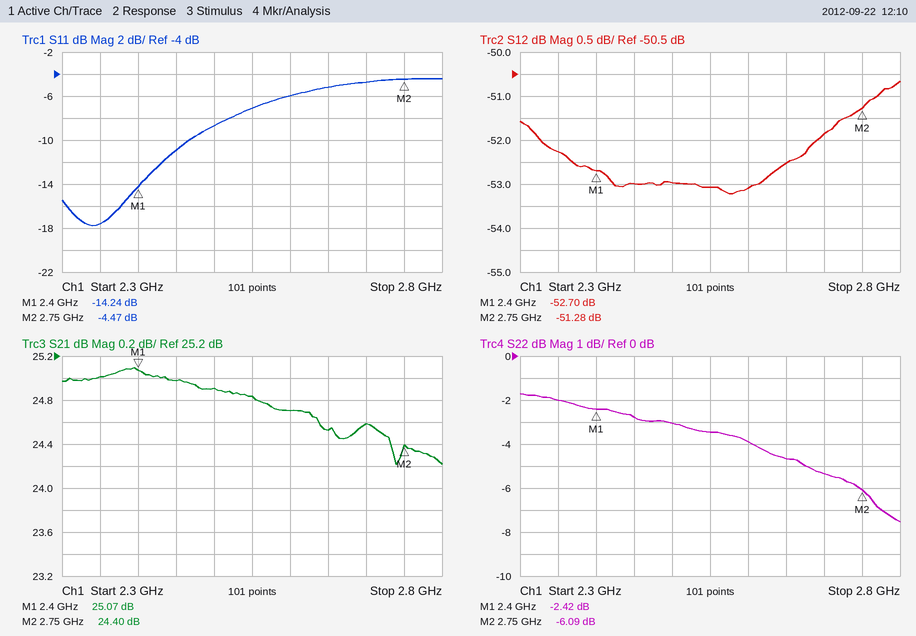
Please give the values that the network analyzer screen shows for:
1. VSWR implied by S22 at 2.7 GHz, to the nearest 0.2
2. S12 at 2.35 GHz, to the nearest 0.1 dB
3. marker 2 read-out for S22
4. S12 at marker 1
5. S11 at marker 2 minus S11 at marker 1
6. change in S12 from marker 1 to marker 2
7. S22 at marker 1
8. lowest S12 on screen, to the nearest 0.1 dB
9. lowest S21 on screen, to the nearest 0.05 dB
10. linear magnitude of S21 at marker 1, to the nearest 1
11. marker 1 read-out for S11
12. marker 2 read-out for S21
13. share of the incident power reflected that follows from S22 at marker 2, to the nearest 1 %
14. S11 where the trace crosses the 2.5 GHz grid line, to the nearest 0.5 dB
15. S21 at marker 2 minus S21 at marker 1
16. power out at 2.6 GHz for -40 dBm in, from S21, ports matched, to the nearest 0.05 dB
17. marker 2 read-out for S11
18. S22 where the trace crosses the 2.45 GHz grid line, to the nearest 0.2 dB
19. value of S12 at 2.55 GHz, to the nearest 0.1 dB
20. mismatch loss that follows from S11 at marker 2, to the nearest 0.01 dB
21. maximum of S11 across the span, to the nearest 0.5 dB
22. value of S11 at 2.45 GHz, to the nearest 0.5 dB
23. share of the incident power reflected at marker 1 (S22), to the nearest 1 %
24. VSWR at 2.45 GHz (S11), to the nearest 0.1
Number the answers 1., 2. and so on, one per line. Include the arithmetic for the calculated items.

1. |Γ| = 10^(-5.4/20) = 0.5370; VSWR = (1 + 0.5370)/(1 − 0.5370) ≈ 3.32, so 3.4 to the nearest 0.2
2. -52.3 dB
3. -6.09 dB
4. -52.70 dB
5. -4.47 − (-14.24) = 9.77 dB
6. -51.28 − (-52.7) = 1.42 dB
7. -2.42 dB
8. -53.2 dB
9. 24.20 dB
10. 10^(25.07/20) ≈ 18
11. -14.24 dB
12. 24.40 dB
13. 10^(-6.09/10) ≈ 25 %
14. -8.5 dB
15. 24.4 − (25.07) = -0.67 dB
16. -40 dBm + (24.70 dB) = -15.30 dBm
17. -4.47 dB
18. -2.8 dB
19. -53.1 dB
20. −10 log10(1 − 10^(-4.47/10)) ≈ 1.92 dB
21. -4.5 dB
22. -11.0 dB
23. 10^(-2.42/10) ≈ 57 %
24. |Γ| = 10^(-11/20) = 0.2818; VSWR = (1 + 0.2818)/(1 − 0.2818) ≈ 1.8
